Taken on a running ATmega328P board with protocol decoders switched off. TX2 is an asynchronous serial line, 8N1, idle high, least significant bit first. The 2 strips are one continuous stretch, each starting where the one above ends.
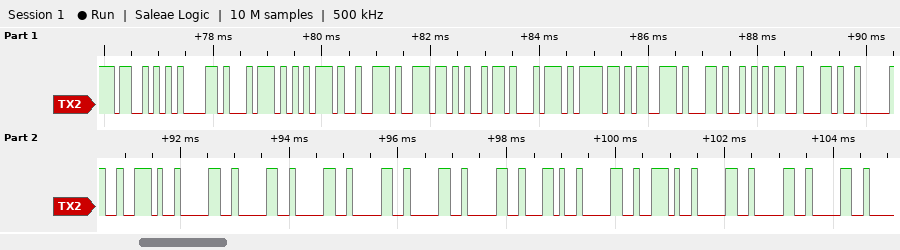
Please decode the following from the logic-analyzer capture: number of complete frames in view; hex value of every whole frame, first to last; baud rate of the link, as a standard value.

27
0x53 0x61 0x74 0x75 0x72 0x6E 0x69 0x74 0x6F 0x73 0x2C 0x35 0x2C 0x30 0x2E 0x30 0x30 0x30 0x30 0x30 0x30 0x2C 0x30 0x2E 0x30 0x30 0x30
9600 baud
